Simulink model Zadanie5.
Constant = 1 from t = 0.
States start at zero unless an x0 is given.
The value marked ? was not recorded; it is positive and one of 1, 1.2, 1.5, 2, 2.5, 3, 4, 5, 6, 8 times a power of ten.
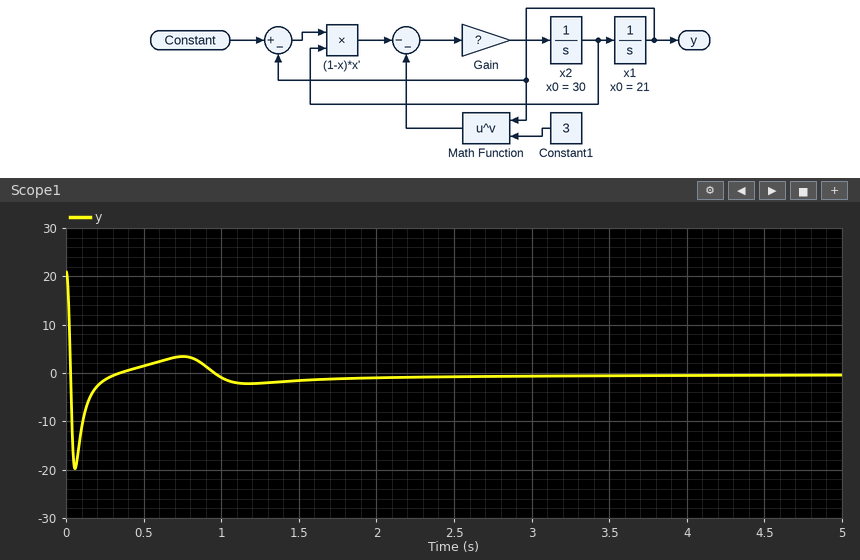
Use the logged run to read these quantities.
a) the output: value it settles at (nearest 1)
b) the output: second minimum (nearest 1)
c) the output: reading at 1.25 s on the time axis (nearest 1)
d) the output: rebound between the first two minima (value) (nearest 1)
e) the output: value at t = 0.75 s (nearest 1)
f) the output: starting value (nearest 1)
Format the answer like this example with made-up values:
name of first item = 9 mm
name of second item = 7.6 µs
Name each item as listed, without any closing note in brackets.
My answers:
the output: value it settles at = 0
the output: second minimum = -2
the output: reading at 1.25 s on the time axis = -2
the output: rebound between the first two minima (value) = 3
the output: value at t = 0.75 s = 3
the output: starting value = 21
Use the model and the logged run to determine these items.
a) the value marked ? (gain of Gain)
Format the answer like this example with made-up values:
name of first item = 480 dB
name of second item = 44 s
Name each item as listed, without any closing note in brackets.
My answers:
the value marked ? = 4
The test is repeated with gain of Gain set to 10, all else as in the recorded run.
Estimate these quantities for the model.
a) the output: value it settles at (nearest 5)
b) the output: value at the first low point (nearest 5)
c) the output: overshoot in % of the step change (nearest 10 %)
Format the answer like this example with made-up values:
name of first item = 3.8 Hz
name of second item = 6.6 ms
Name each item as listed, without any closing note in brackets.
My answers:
the output: value it settles at = 0
the output: value at the first low point = -20
the output: overshoot in % of the step change = 90 %
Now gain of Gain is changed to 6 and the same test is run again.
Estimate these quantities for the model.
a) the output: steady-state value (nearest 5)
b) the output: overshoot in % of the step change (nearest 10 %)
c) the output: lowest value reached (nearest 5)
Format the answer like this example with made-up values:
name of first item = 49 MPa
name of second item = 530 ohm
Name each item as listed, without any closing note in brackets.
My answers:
the output: steady-state value = 0
the output: overshoot in % of the step change = 90 %
the output: lowest value reached = -20
